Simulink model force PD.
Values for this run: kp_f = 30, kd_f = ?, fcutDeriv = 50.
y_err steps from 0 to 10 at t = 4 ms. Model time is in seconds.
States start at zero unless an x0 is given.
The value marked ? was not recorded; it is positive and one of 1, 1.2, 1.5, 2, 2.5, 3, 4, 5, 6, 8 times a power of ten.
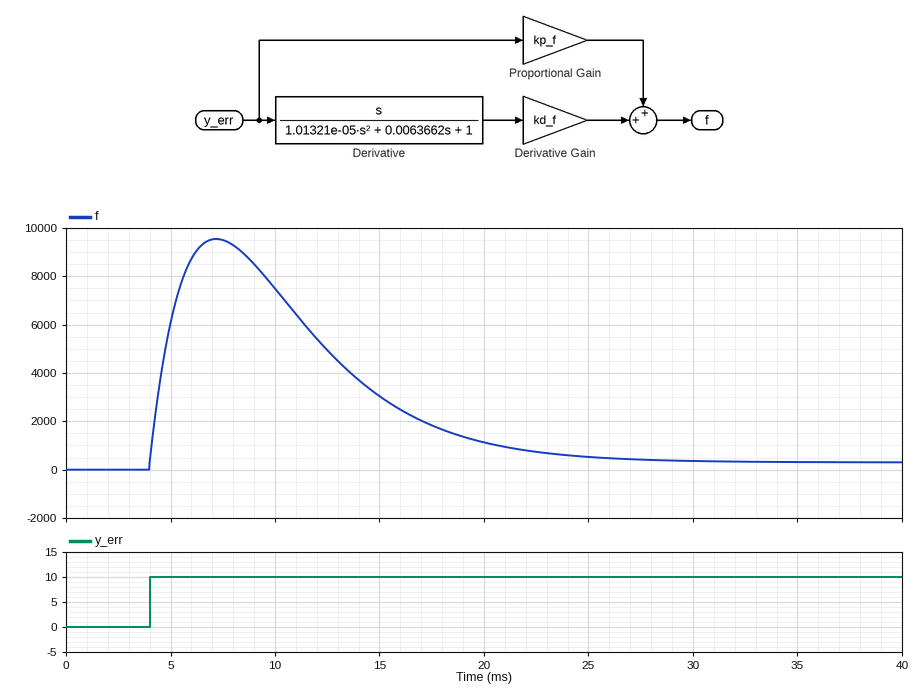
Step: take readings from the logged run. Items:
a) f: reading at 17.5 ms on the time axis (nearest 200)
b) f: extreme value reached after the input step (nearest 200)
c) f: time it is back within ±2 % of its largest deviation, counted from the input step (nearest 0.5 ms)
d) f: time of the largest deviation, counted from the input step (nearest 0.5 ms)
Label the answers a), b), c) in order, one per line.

a) 1800
b) 9600
c) 21.5 ms
d) 3.0 ms
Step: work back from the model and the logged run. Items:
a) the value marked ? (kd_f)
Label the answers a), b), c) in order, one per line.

a) 8
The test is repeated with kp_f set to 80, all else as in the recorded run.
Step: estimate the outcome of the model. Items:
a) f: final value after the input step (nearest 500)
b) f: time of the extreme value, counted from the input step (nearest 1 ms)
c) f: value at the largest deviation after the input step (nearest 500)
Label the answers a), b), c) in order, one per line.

a) 1000
b) 3 ms
c) 10000
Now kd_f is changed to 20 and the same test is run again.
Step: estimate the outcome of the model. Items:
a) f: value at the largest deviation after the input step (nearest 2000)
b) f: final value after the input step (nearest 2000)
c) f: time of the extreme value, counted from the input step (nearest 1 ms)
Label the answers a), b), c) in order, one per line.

a) 24000
b) 0
c) 3 ms
